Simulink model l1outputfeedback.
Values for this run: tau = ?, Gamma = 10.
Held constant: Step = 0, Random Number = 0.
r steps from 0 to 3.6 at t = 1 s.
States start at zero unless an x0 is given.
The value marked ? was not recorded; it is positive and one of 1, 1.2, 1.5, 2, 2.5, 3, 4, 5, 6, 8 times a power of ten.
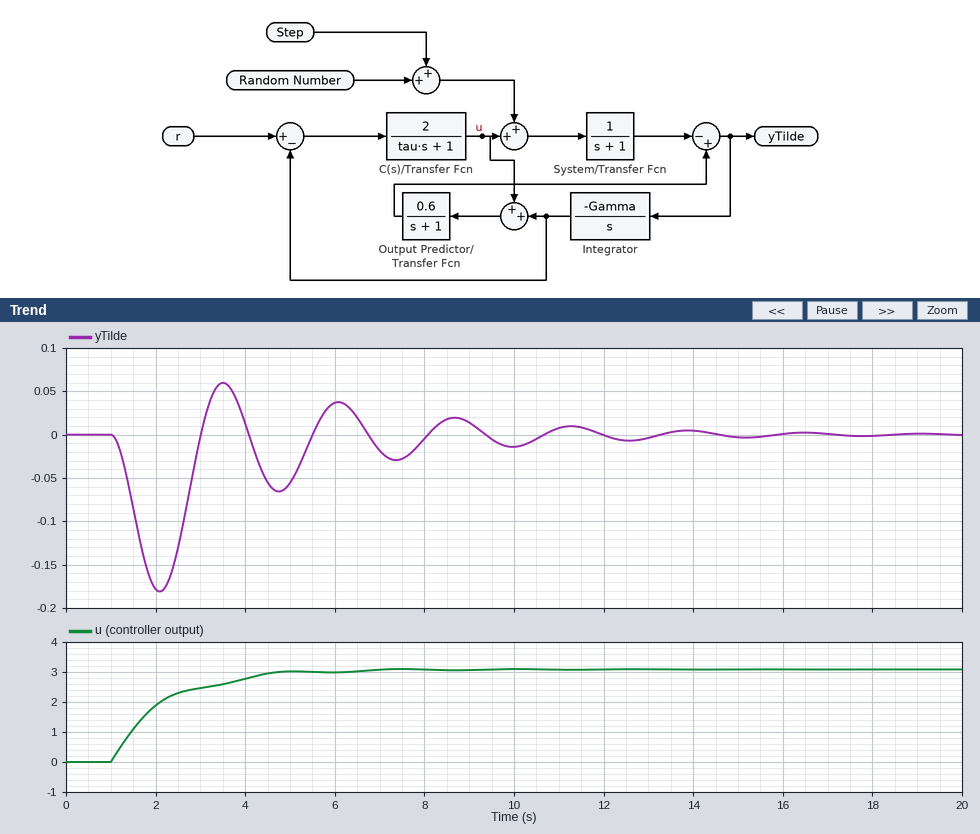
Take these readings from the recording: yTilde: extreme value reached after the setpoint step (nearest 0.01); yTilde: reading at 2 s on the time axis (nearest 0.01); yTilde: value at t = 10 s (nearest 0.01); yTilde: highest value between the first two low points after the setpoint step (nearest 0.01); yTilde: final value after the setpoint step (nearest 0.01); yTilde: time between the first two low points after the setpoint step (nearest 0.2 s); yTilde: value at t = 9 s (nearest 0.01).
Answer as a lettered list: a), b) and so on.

a) -0.18
b) -0.18
c) -0.01
d) 0.06
e) 0.00
f) 2.6 s
g) 0.01
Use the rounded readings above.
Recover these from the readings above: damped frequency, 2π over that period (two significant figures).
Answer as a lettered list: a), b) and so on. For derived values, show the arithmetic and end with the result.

a) 2π / 2.6 = 2.4 rad/s
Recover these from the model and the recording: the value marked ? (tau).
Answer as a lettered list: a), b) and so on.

a) 3
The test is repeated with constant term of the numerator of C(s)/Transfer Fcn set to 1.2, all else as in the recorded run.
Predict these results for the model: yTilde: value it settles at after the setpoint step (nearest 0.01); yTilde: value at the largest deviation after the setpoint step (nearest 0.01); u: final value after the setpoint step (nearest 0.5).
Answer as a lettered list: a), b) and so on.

a) 0.00
b) -0.11
c) 2.5
